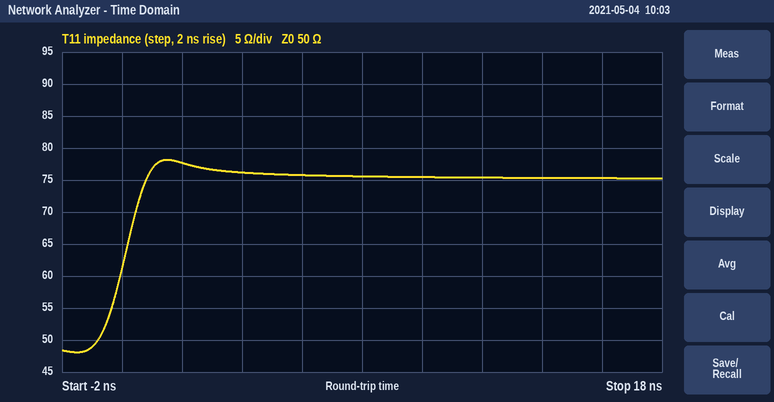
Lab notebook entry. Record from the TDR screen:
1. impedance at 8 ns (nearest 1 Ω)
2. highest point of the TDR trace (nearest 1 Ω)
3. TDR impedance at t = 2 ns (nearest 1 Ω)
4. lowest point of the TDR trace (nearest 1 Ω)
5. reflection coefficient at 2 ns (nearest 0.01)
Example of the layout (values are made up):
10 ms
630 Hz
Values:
76 Ω
78 Ω
78 Ω
48 Ω
+0.22
